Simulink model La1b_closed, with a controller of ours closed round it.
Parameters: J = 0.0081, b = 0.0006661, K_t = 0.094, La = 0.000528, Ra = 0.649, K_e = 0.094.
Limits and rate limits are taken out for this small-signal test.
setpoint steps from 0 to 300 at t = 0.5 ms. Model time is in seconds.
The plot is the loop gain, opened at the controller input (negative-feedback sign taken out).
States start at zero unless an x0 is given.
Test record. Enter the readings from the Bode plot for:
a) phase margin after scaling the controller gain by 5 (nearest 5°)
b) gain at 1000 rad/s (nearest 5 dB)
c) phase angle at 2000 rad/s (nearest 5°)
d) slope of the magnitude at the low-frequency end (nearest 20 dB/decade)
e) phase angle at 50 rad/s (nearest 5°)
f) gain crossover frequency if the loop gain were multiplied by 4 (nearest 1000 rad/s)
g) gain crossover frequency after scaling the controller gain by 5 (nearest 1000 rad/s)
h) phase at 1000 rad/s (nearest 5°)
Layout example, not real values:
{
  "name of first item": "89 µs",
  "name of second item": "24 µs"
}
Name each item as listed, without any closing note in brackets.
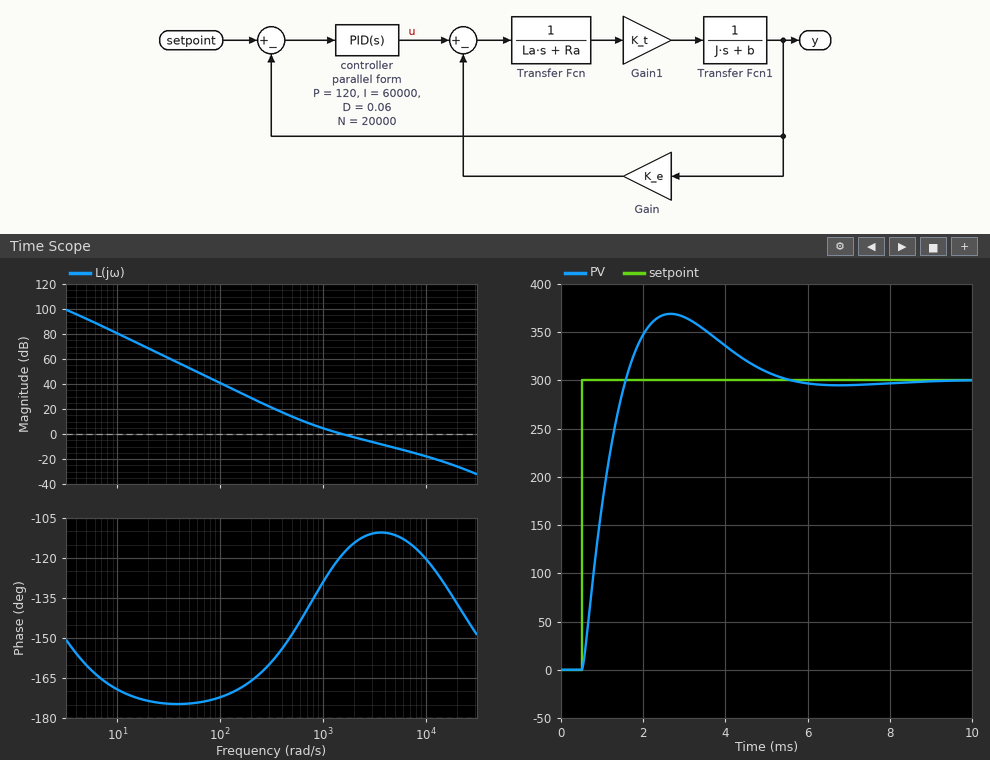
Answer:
{
  "phase margin after scaling the controller gain by 5": "65°",
  "gain at 1000 rad/s": "5 dB",
  "phase angle at 2000 rad/s": "-115°",
  "slope of the magnitude at the low-frequency end": "-40 dB/decade",
  "phase angle at 50 rad/s": "-175°",
  "gain crossover frequency if the loop gain were multiplied by 4": "6000 rad/s",
  "gain crossover frequency after scaling the controller gain by 5": "7000 rad/s",
  "phase at 1000 rad/s": "-130°"
}
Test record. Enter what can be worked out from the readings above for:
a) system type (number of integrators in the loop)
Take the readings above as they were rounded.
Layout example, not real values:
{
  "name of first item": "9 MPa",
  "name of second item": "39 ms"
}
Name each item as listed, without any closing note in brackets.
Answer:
{
  "system type": "2"
}
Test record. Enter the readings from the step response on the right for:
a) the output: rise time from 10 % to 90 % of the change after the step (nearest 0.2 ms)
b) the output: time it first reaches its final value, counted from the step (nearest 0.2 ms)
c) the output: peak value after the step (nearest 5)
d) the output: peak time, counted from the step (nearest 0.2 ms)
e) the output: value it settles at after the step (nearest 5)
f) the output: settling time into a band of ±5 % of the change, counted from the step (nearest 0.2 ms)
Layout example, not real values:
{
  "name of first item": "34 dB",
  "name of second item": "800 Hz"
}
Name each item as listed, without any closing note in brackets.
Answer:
{
  "the output: rise time from 10 % to 90 % of the change after the step": "0.8 ms",
  "the output: time it first reaches its final value, counted from the step": "1.0 ms",
  "the output: peak value after the step": "370",
  "the output: peak time, counted from the step": "2.2 ms",
  "the output: value it settles at after the step": "300",
  "the output: settling time into a band of ±5 % of the change, counted from the step": "4.2 ms"
}
